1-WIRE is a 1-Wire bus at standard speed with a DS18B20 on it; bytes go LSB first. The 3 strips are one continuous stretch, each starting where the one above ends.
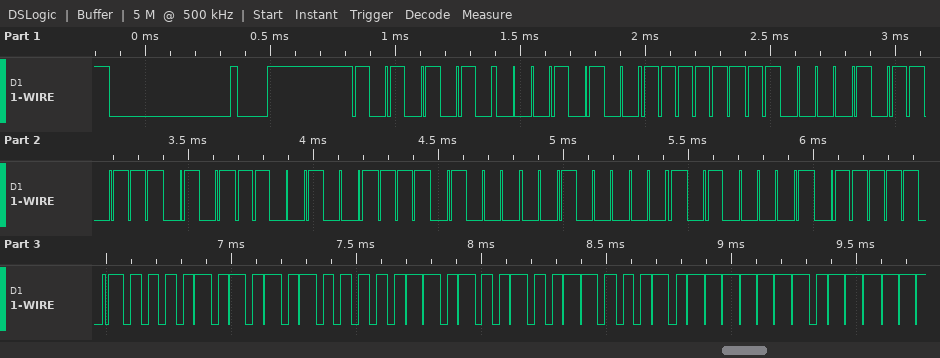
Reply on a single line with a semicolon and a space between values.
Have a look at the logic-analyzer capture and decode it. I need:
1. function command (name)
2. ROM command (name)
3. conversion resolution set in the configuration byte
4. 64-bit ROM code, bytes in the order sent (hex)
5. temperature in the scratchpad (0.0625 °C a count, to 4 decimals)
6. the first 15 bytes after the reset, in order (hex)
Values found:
Read Scratchpad; Match ROM; 12 bits; 28 FF D0 AE 93 17 04 85; 85.0000 °C; 55 28 FF D0 AE 93 17 04 85 BE 50 05 4B 46 7F
